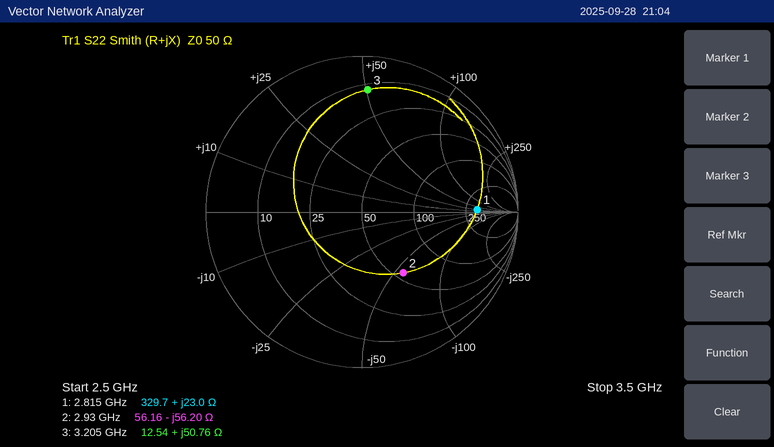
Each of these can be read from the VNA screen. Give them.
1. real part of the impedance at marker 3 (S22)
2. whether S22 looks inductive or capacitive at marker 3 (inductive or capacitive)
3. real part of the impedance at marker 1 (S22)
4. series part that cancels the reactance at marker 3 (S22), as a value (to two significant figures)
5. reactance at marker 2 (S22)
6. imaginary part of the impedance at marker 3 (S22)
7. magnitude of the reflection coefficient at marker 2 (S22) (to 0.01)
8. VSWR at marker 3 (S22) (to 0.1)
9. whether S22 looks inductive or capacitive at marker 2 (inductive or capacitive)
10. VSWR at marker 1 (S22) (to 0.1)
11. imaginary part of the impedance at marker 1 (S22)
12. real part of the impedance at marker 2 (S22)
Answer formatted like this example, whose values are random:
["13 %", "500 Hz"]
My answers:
["12.54 Ω", "inductive", "329.7 Ω", "980 fF", "-56.20 Ω", "+50.76 Ω", "0.47", "8.2", "capacitive", "6.6", "+23.0 Ω", "56.16 Ω"]
